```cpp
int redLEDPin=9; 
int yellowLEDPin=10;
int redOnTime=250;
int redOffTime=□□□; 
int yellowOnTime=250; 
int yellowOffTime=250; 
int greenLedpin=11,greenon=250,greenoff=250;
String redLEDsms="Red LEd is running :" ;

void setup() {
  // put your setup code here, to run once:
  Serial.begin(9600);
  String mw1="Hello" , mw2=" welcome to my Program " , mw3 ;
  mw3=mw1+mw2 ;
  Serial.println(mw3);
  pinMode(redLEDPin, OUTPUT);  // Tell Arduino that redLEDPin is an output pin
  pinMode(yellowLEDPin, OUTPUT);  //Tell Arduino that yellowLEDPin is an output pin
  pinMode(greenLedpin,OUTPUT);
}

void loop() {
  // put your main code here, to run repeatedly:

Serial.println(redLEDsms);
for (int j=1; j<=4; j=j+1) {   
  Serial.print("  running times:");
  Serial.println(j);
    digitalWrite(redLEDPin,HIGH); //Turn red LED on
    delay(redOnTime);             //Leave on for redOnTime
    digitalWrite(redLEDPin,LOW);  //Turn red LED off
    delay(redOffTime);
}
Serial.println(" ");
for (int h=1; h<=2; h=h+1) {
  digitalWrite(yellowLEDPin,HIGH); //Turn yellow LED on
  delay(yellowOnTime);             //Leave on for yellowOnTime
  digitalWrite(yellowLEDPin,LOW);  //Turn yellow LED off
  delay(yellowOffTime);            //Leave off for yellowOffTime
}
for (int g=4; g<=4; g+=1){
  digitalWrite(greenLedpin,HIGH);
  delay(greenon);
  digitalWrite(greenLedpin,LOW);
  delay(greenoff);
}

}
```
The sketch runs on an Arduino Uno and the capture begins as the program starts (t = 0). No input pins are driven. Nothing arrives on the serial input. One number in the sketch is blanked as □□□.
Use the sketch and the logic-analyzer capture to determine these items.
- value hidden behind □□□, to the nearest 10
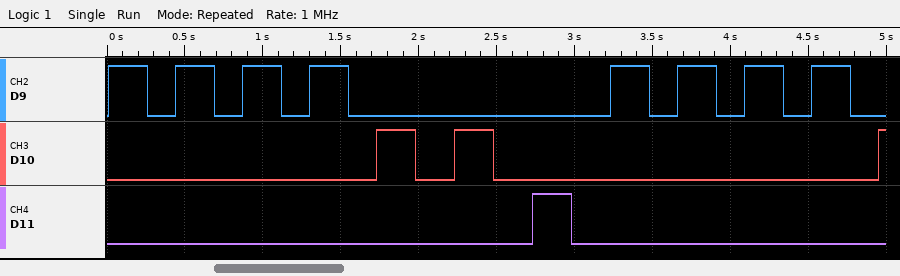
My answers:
180
